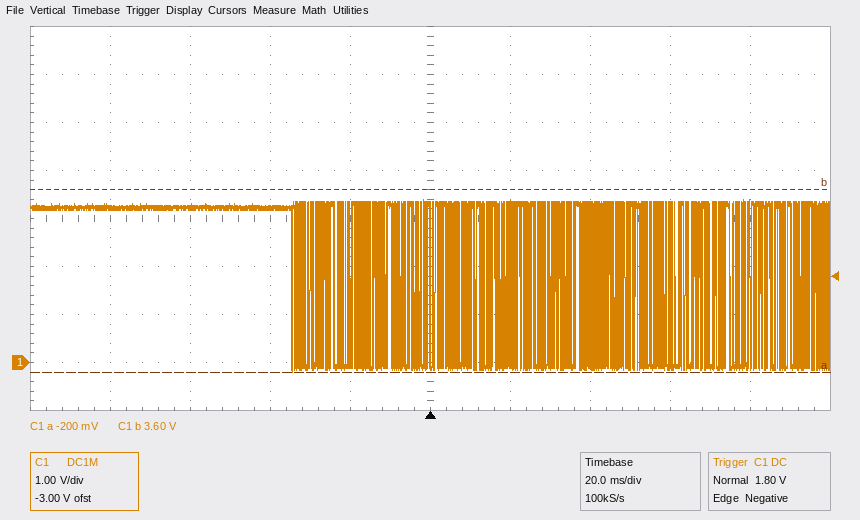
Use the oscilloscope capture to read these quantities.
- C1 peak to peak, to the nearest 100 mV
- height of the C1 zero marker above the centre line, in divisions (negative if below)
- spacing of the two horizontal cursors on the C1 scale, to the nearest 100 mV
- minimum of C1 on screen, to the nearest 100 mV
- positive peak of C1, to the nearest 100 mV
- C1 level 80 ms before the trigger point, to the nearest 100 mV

3.6 V
-3.0 div
3.8 V
-200 mV
3.4 V
3.2 V
